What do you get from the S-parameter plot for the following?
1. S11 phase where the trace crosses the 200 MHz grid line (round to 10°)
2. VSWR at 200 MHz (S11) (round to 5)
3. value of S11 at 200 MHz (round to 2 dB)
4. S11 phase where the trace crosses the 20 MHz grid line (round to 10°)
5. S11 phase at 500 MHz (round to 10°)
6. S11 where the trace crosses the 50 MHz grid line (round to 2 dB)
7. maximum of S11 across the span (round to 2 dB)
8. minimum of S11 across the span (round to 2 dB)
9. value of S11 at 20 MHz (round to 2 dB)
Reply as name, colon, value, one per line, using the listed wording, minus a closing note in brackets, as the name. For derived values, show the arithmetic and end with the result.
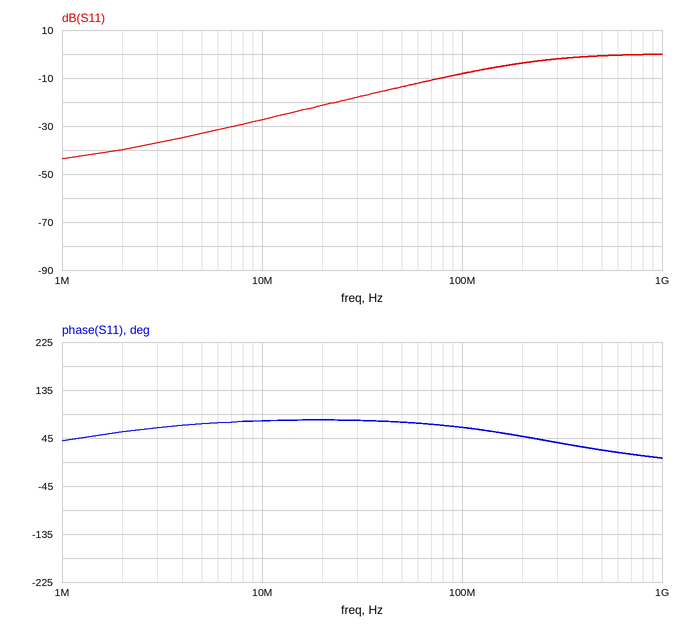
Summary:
S11 phase where the trace crosses the 200 MHz grid line: 50°
VSWR at 200 MHz (S11): |Γ| = 10^(-4/20) = 0.6310; VSWR = (1 + 0.6310)/(1 − 0.6310) ≈ 4.42, so 5 to the nearest 5
value of S11 at 200 MHz: -4 dB
S11 phase where the trace crosses the 20 MHz grid line: 80°
S11 phase at 500 MHz: 20°
S11 where the trace crosses the 50 MHz grid line: -14 dB
maximum of S11 across the span: 0 dB
minimum of S11 across the span: -44 dB
value of S11 at 20 MHz: -22 dB
